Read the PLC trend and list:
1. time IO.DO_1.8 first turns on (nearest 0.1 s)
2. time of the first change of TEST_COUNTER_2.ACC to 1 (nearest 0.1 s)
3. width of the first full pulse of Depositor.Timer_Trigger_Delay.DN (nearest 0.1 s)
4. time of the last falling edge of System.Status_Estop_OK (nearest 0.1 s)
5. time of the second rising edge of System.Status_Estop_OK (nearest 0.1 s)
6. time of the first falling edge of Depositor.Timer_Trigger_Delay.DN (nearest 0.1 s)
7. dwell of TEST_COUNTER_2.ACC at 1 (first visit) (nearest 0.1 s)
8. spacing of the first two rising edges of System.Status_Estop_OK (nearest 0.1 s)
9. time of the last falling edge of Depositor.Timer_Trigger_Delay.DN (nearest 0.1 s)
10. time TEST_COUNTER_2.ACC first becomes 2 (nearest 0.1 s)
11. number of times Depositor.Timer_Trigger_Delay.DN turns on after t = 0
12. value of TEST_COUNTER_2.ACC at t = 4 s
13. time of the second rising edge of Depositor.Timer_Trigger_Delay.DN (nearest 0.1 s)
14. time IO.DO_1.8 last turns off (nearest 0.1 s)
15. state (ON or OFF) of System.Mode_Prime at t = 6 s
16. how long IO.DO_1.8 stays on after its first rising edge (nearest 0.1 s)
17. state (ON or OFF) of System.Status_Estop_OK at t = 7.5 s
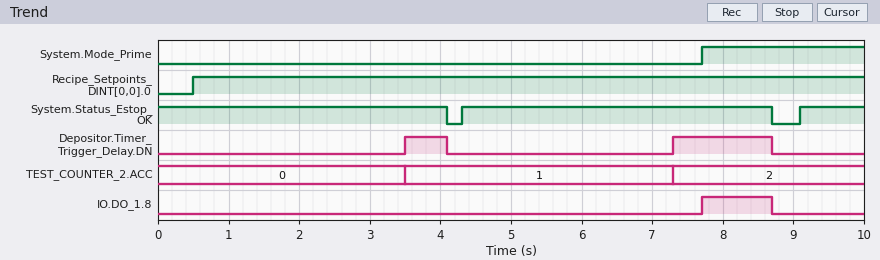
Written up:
7.7 s
3.5 s
0.6 s
8.7 s
9.1 s
4.1 s
3.8 s
4.8 s
8.7 s
7.3 s
2
1
7.3 s
8.7 s
OFF
1.0 s
ON
